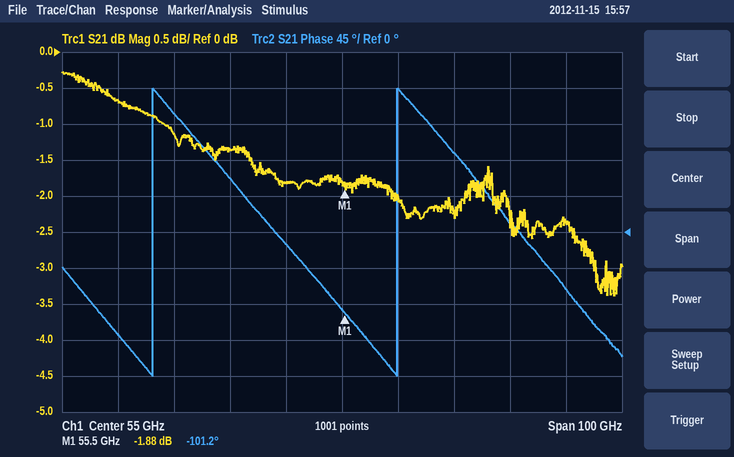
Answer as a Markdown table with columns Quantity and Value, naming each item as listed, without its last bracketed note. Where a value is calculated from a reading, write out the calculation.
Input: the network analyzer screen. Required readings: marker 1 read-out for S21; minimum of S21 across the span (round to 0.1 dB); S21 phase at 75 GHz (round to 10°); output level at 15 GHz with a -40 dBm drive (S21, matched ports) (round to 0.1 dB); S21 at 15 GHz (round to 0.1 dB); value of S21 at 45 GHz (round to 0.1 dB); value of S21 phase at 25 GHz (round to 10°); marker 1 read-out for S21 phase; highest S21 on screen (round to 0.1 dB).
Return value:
| Quantity | Value |
|---|---|
| marker 1 read-out for S21 | -1.88 dB |
| minimum of S21 across the span | -3.4 dB |
| S21 phase at 75 GHz | 100° |
| output level at 15 GHz with a -40 dBm drive (S21, matched ports) | -40 dBm + (-0.7 dB) = -40.7 dBm |
| S21 at 15 GHz | -0.7 dB |
| value of S21 at 45 GHz | -1.8 dB |
| value of S21 phase at 25 GHz | 150° |
| marker 1 read-out for S21 phase | -101.2° |
| highest S21 on screen | -0.3 dB |
